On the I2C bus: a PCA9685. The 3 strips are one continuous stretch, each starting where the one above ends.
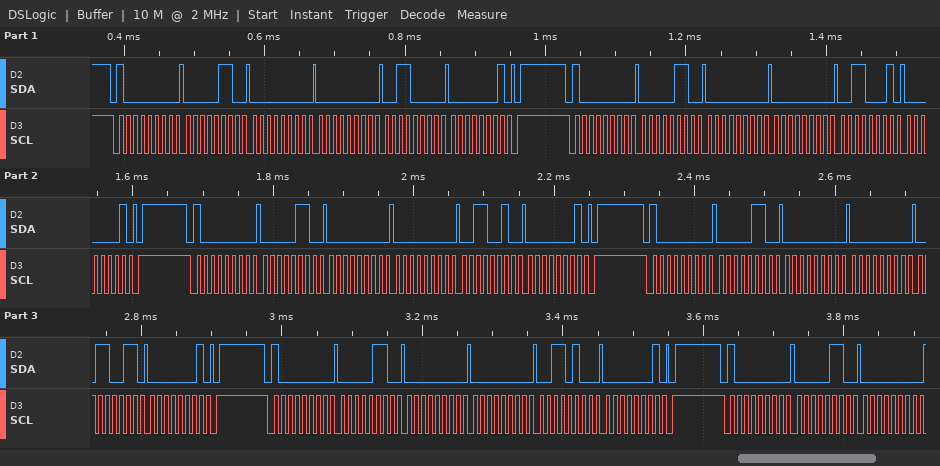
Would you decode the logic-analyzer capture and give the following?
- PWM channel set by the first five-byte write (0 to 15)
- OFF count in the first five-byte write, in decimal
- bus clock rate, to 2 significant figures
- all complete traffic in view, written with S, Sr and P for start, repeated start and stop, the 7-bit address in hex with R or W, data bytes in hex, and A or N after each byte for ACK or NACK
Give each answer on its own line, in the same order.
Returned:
0
304
100 kHz
S 40W A 06 A 00 A 00 A 30 A 01 A P S 40W A 06 A 00 A 00 A 31 A 01 A P S 40W A 06 A 00 A 00 A 32 A 01 A P S 40W A 06 A 00 A 00 A 33 A 01 A P S 40W A 06 A 00 A 00 A 34 A 01 A P S 40W A 06 A 00 A
